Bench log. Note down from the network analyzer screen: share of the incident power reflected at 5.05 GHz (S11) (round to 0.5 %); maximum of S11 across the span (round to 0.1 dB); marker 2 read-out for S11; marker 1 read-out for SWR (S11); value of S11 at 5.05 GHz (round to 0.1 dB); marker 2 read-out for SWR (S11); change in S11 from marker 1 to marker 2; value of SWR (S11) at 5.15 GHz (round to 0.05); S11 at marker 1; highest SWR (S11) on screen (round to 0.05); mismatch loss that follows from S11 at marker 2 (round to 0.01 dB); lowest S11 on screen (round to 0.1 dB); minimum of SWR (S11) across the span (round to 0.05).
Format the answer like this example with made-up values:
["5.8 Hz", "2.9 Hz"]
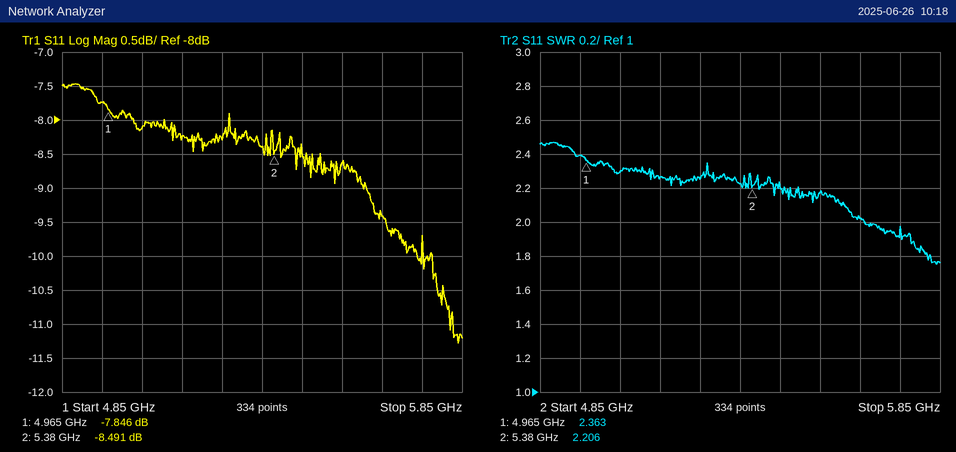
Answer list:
["15.5 %", "-7.5 dB", "-8.491 dB", "2.363", "-8.1 dB", "2.206", "-0.645 dB", "2.25", "-7.846 dB", "2.45", "0.66 dB", "-11.3 dB", "1.75"]
